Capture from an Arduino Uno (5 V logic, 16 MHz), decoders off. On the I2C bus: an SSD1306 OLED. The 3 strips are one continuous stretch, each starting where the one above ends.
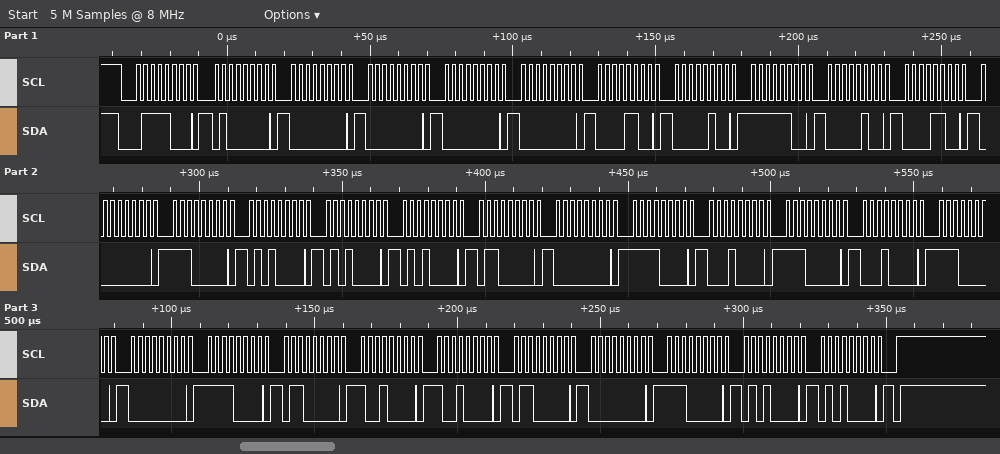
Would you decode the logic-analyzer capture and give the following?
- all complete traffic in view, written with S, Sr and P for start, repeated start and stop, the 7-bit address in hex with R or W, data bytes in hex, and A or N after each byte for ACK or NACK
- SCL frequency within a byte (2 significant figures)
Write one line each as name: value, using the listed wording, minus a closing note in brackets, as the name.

all complete traffic in view, written with S, Sr and P for start, repeated start and stop, the 7-bit address in hex with R or W, data bytes in hex, and A or N after each byte for ACK or NACK: S 3CW A 40 A 00 A 00 A 00 A 00 A 0C A 04 A FC A 04 A 0C A 00 A E0 A 50 A 50 A 50 A 60 A 00 A F0 A 10 A E0 A 10 A E0 A 00 A F0 A 60 A 90 A 90 A 60 A 00 A E0 A 50 A 50 A P
SCL frequency within a byte: 400 kHz
